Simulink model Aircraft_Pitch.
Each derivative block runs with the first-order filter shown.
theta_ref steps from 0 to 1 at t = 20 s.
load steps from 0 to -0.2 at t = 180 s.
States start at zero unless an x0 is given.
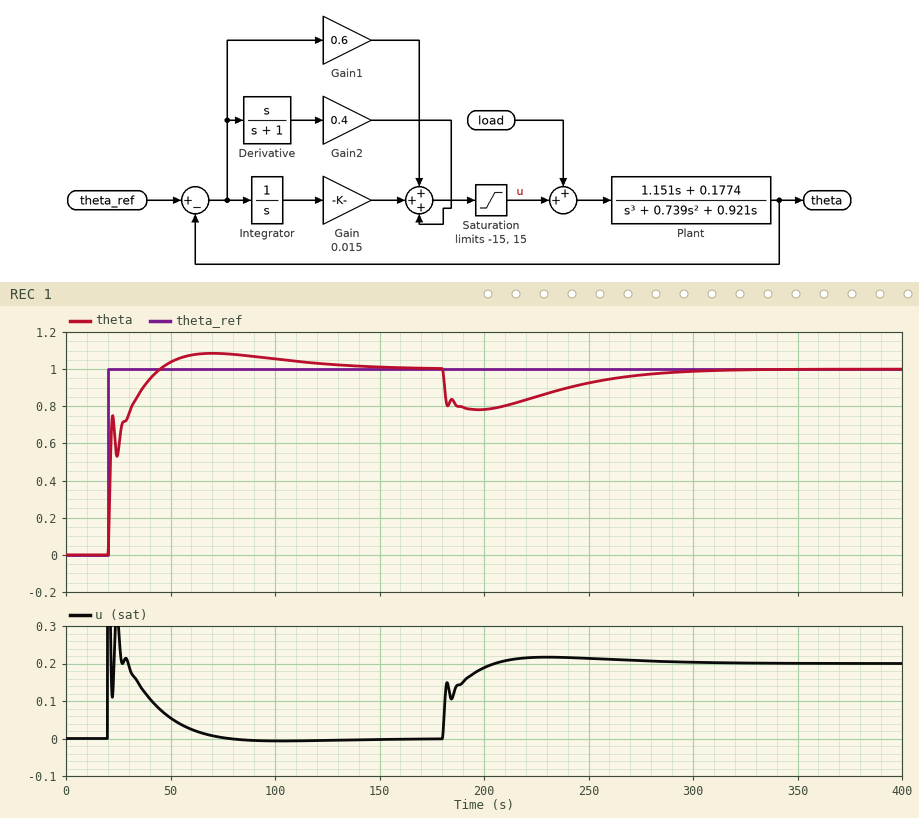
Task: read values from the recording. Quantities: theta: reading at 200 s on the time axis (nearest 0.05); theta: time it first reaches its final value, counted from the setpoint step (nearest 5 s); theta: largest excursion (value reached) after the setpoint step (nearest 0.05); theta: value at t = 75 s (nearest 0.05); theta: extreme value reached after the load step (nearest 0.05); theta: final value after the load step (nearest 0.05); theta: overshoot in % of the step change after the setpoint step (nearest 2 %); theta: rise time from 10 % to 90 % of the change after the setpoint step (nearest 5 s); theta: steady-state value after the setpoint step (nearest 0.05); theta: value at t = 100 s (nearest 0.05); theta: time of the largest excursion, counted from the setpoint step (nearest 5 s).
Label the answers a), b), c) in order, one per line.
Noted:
a) 0.80
b) 25 s
c) 1.10
d) 1.10
e) 0.80
f) 1.00
g) 8 %
h) 15 s
i) 1.00
j) 1.05
k) 50 s
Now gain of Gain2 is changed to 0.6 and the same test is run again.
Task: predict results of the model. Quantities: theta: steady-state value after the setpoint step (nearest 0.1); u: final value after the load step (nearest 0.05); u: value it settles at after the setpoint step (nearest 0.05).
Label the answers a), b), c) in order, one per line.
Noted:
a) 1.0
b) 0.20
c) 0.00
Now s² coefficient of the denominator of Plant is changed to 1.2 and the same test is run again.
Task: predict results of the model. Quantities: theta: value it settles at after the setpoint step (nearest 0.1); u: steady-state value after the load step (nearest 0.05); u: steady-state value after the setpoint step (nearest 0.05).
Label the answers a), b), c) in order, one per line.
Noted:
a) 1.0
b) 0.20
c) 0.00
